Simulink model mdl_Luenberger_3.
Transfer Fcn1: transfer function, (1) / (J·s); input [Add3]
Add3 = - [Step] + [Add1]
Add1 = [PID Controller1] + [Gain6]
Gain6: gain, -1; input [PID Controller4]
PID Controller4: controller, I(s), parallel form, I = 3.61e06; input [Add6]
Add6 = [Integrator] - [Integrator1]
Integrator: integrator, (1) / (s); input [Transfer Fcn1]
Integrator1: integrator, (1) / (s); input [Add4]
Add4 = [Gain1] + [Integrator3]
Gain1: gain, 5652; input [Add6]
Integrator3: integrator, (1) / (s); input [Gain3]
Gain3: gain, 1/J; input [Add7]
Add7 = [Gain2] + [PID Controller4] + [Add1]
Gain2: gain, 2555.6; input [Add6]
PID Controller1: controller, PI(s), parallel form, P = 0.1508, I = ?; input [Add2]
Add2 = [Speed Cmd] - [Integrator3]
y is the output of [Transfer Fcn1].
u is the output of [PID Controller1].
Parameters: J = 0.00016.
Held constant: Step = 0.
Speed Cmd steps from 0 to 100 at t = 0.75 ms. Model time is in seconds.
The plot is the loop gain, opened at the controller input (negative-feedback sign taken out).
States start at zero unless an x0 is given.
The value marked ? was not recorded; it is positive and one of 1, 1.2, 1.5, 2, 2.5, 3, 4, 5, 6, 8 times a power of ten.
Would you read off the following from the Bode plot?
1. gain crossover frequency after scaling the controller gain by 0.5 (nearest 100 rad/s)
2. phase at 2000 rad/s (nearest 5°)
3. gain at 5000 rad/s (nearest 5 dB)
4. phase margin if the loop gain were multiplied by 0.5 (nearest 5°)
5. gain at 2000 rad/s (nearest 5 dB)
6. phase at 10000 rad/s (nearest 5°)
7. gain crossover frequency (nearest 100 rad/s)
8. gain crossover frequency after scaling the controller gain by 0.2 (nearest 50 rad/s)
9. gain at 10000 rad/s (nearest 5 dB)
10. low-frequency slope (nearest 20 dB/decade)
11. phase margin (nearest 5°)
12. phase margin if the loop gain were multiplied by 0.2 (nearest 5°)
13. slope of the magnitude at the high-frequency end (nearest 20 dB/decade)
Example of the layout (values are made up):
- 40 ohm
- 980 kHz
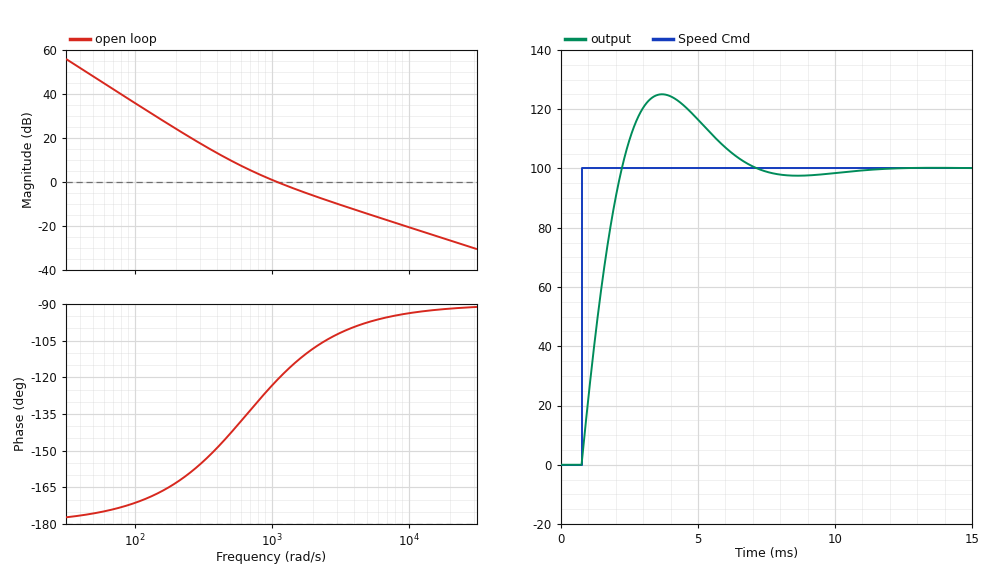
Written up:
- 700 rad/s
- -110°
- -15 dB
- 45°
- -5 dB
- -95°
- 1100 rad/s
- 400 rad/s
- -20 dB
- -40 dB/decade
- 60°
- 30°
- -20 dB/decade
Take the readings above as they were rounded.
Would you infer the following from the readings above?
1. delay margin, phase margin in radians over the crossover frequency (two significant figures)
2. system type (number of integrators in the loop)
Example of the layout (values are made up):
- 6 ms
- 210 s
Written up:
- 0.00095 s
- 2
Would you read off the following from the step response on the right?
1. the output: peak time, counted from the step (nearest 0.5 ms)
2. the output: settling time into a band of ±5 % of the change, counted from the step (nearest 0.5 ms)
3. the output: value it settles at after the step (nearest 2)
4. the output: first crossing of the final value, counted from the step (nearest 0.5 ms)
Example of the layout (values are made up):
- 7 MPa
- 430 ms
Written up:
- 3.0 ms
- 5.5 ms
- 100
- 1.5 ms
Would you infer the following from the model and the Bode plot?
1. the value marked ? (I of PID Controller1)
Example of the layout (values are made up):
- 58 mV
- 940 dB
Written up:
- 100
